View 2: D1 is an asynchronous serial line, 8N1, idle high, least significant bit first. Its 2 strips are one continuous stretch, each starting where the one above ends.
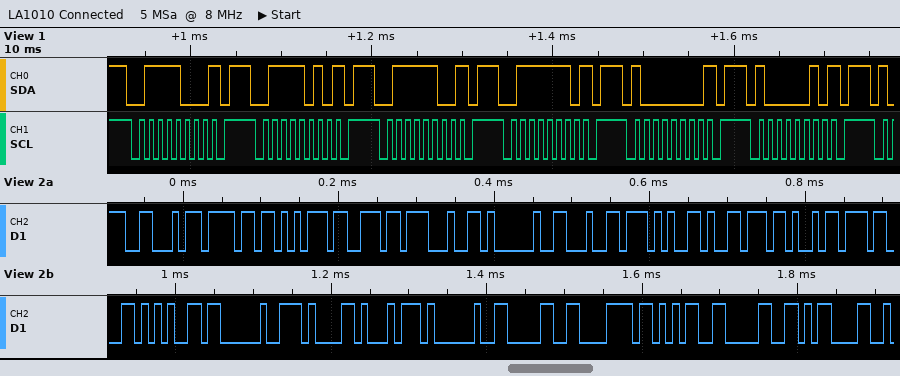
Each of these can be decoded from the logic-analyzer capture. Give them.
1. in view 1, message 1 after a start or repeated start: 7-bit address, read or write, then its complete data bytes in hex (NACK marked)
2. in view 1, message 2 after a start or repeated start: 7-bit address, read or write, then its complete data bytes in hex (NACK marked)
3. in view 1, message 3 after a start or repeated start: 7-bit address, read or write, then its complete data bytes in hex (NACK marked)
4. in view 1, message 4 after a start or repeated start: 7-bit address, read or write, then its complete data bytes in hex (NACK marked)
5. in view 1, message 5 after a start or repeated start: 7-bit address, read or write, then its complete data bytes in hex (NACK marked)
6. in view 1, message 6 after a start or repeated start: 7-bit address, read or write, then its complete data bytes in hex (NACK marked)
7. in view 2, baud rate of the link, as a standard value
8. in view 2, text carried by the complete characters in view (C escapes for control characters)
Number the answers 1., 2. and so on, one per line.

1. 0x3C write NACK
2. 0x3D write NACK
3. 0x3E write NACK
4. 0x3F write NACK
5. 0x40 write NACK
6. 0x41 write NACK
7. 115200 baud
8. "Found device at 0x50\r"
